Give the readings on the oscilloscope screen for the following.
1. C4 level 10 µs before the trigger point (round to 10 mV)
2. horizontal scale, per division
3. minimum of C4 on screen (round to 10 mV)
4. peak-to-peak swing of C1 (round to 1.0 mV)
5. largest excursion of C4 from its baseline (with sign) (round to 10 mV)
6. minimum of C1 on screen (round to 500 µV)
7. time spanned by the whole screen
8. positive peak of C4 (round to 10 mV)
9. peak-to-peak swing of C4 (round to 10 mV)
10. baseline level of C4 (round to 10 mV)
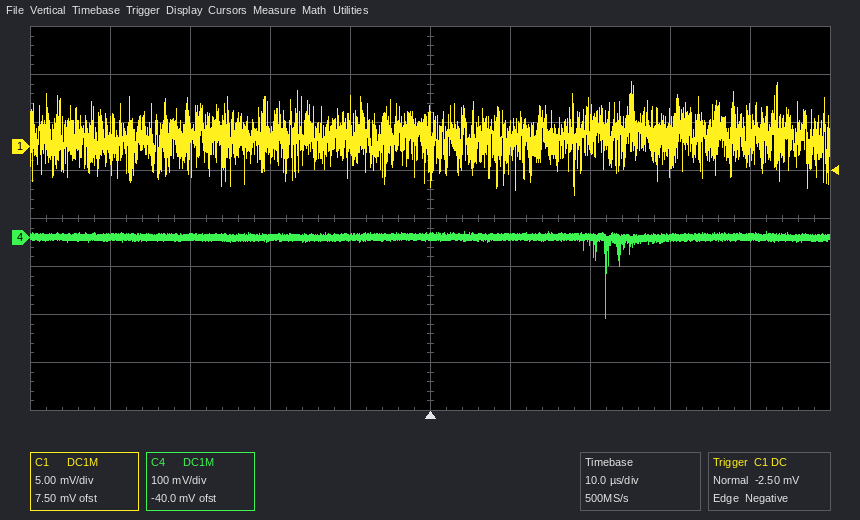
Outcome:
0 mV
10 µs
-170 mV
12.0 mV
-170 mV
-5.0 mV
100 µs
10 mV
180 mV
0 mV
